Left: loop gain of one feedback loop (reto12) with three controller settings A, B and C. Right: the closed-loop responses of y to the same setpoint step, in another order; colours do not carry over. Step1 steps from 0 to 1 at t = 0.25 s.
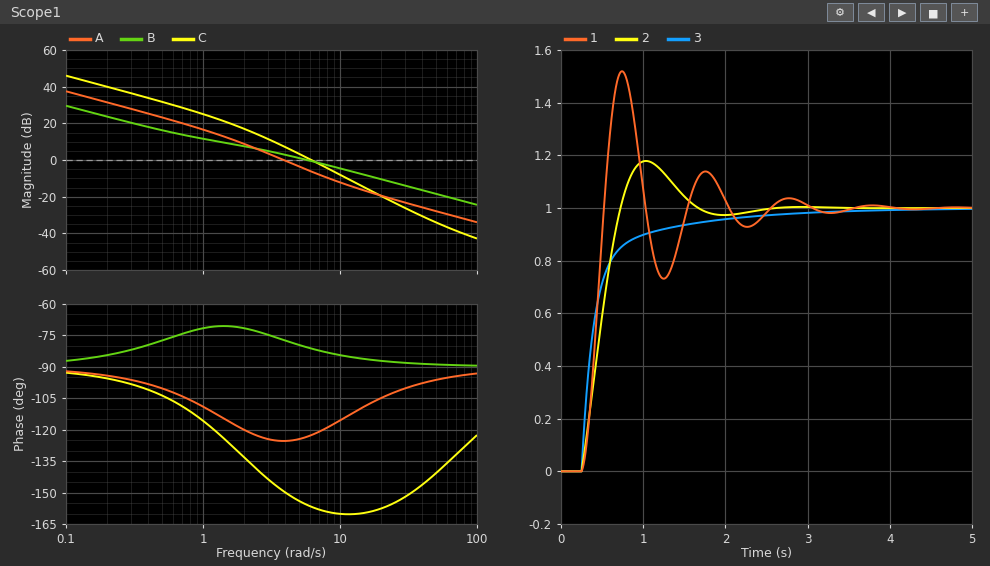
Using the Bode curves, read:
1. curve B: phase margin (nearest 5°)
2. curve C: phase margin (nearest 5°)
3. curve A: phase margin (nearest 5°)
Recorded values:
100°
25°
55°
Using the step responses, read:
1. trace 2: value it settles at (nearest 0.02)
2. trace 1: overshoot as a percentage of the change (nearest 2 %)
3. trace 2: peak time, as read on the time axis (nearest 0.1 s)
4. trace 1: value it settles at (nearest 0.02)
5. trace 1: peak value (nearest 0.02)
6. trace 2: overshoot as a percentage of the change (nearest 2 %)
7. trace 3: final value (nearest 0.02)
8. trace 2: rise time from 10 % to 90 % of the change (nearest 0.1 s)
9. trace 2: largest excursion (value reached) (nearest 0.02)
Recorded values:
1.00
52 %
1.0 s
1.00
1.52
18 %
1.00
0.4 s
1.18
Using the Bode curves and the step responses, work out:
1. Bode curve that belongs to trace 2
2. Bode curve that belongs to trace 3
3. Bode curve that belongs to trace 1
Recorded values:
A
B
C
